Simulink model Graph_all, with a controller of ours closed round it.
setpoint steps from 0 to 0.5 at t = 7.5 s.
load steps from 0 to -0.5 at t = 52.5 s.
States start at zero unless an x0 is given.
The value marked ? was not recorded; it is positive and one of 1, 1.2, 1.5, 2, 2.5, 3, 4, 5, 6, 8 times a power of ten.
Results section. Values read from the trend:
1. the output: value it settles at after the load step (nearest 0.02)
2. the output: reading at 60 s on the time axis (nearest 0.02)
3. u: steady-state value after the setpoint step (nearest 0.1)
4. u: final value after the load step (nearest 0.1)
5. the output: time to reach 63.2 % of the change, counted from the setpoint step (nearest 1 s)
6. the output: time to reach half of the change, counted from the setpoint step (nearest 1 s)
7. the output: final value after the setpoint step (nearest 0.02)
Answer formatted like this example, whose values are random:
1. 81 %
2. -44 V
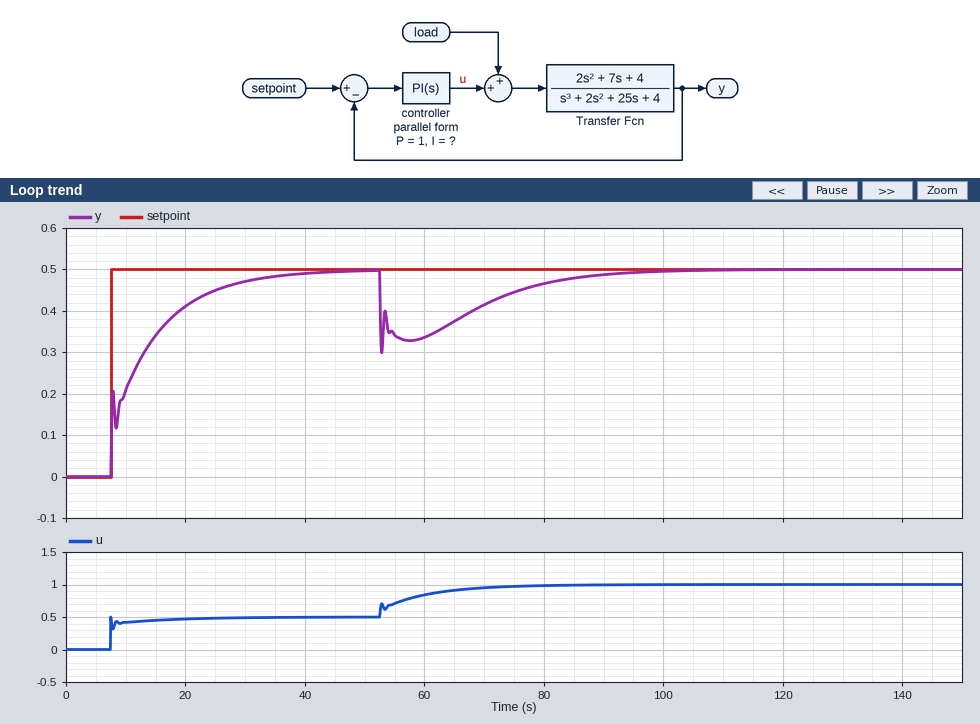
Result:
1. 0.50
2. 0.34
3. 0.5
4. 1.0
5. 6 s
6. 4 s
7. 0.50
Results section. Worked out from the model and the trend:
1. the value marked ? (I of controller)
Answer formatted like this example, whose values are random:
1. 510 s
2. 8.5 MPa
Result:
1. 0.15
